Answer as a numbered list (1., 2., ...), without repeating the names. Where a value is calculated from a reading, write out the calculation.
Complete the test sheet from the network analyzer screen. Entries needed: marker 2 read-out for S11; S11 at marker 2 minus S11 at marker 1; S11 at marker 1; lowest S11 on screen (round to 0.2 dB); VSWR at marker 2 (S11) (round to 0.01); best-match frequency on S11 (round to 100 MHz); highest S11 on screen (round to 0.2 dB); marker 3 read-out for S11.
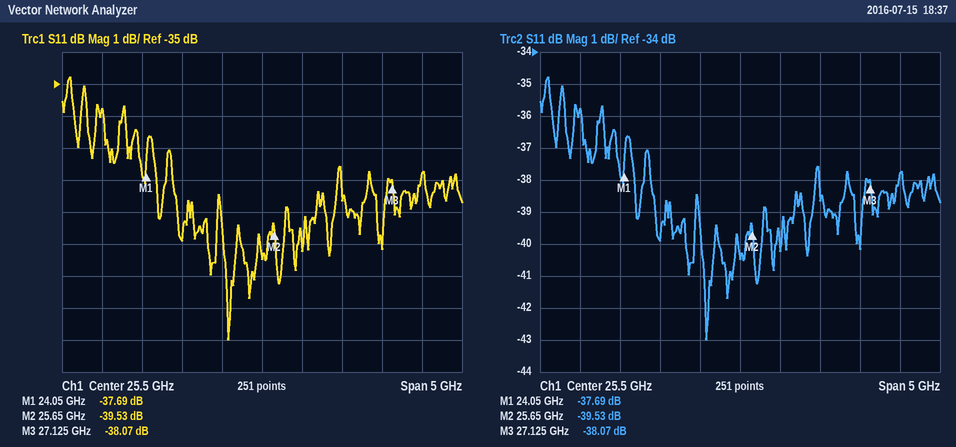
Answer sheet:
1. -39.53 dB
2. -39.53 − (-37.69) = -1.84 dB
3. -37.69 dB
4. -43.0 dB
5. (1 + 0.0106)/(1 − 0.0106) ≈ 1.02
6. 25.1 GHz
7. -34.8 dB
8. -38.07 dB
